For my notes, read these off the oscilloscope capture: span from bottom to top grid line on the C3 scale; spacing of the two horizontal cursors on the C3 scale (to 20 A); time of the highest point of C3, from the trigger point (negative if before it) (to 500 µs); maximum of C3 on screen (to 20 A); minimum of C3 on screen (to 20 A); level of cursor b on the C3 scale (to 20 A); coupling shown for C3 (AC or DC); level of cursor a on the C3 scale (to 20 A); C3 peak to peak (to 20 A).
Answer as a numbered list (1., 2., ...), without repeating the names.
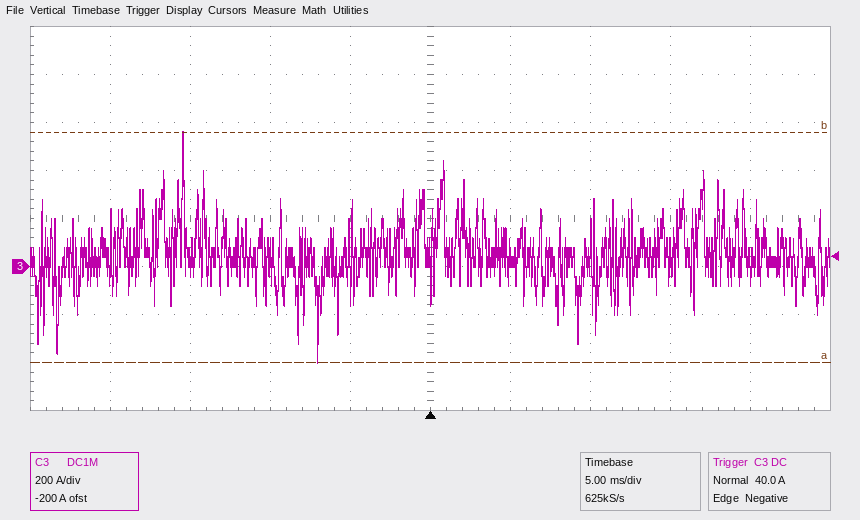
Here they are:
1. 1.6 kA
2. 960 A
3. -15.5 ms
4. 560 A
5. -400 A
6. 560 A
7. DC
8. -400 A
9. 960 A
